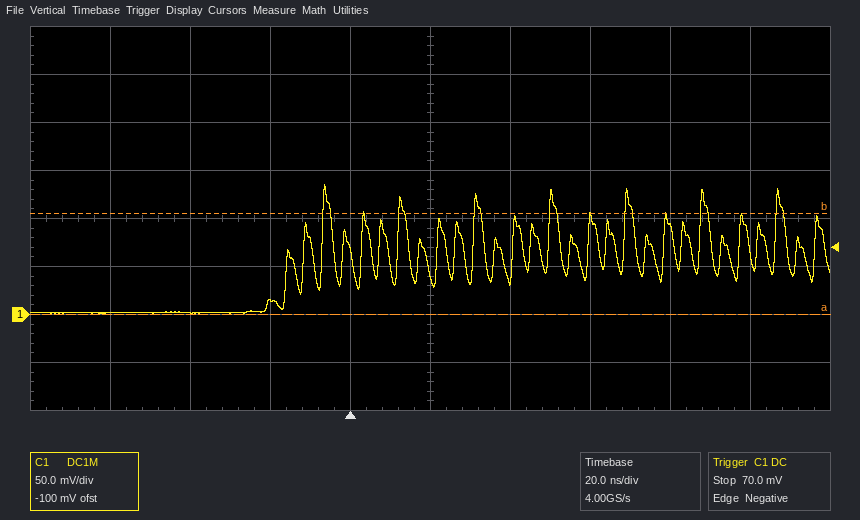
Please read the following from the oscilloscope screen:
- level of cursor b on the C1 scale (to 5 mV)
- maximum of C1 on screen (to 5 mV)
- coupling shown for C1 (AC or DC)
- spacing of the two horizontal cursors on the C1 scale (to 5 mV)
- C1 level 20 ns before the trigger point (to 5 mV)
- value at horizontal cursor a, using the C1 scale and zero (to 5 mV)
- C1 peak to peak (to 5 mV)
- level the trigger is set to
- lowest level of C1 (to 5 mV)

105 mV
135 mV
DC
105 mV
10 mV
0 mV
135 mV
70.0 mV
0 mV
